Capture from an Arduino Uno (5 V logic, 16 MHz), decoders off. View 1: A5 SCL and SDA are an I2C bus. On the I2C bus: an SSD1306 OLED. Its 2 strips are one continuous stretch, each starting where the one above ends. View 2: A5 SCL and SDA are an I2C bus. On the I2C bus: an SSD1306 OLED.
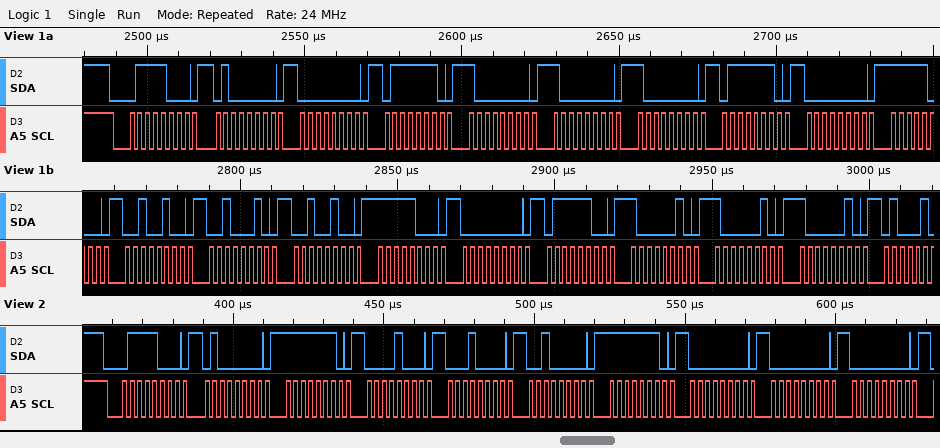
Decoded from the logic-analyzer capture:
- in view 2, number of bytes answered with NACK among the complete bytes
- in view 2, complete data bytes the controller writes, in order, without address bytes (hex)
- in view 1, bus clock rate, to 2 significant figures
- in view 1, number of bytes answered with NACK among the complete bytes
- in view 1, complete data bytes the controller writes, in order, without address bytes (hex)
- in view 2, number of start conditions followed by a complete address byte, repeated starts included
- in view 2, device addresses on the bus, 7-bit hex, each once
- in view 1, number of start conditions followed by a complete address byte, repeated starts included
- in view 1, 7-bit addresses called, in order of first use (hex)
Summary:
0
40 FE 08 10 20 FE 00 00 00
400 kHz
0
40 00 7E 80 80 80 7E 00 F8 24 22 24 F8 00 7C 82 82 82
1
0x3C
1
0x3C
